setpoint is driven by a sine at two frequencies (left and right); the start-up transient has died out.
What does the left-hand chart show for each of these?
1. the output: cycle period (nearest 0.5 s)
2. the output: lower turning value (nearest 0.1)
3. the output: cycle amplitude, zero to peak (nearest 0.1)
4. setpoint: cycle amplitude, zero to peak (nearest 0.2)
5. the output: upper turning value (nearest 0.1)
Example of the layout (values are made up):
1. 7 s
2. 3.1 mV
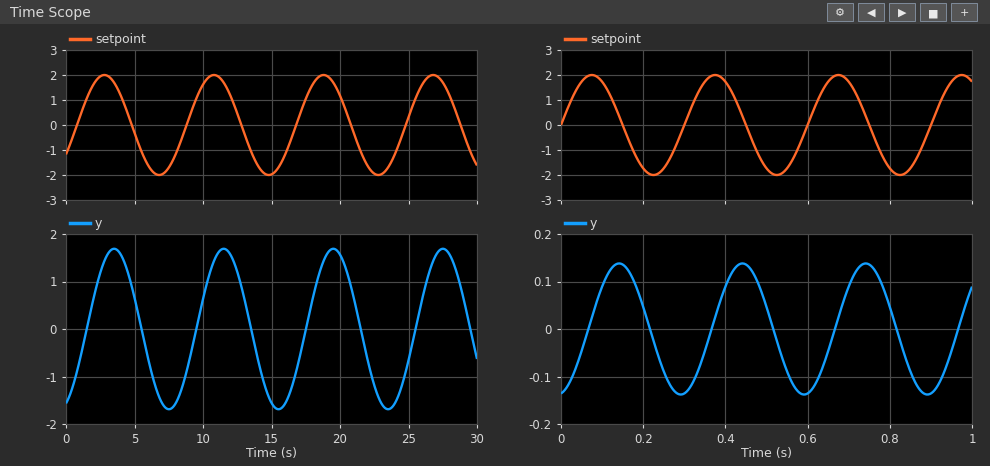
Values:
1. 8.0 s
2. -1.7
3. 1.7
4. 2.0
5. 1.7
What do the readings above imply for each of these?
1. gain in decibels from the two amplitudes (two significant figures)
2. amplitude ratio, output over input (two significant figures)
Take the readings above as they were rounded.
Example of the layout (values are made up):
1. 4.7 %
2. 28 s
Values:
1. -1.4 dB
2. 0.85
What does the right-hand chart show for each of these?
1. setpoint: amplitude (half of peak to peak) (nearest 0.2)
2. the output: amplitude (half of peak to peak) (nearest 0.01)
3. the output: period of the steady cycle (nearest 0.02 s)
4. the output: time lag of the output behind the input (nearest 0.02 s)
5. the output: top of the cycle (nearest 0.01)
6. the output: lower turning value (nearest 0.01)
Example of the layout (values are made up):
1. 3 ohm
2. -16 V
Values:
1. 2.0
2. 0.14
3. 0.30 s
4. 0.06 s
5. 0.14
6. -0.14
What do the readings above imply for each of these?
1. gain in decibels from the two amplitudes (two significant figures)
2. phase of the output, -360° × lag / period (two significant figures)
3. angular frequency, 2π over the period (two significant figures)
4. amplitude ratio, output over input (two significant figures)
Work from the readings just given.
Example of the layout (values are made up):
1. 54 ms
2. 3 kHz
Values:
1. -23 dB
2. -72°
3. 21 rad/s
4. 0.070
